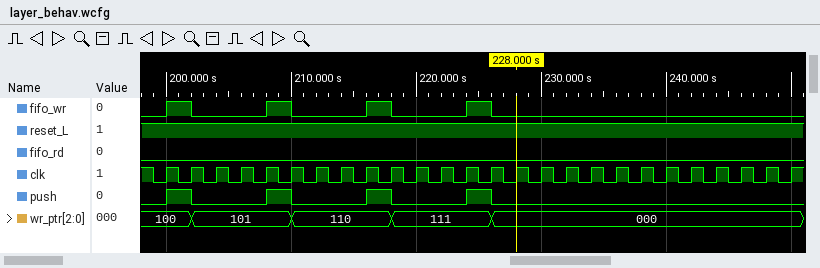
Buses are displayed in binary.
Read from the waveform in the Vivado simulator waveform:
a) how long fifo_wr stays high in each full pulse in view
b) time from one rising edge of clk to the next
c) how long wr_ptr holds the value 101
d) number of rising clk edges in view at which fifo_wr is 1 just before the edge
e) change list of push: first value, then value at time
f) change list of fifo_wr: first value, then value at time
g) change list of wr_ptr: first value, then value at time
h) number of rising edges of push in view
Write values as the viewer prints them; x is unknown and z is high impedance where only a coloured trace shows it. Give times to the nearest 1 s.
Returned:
2 s, 2 s, 2 s, 2 s
2 s
8 s
4
0, 1 at 200 s, 0 at 202 s, 1 at 208 s, 0 at 210 s, 1 at 216 s, 0 at 218 s, 1 at 224 s, 0 at 226 s
0, 1 at 200 s, 0 at 202 s, 1 at 208 s, 0 at 210 s, 1 at 216 s, 0 at 218 s, 1 at 224 s, 0 at 226 s
100, 101 at 202 s, 110 at 210 s, 111 at 218 s, 000 at 226 s
4
